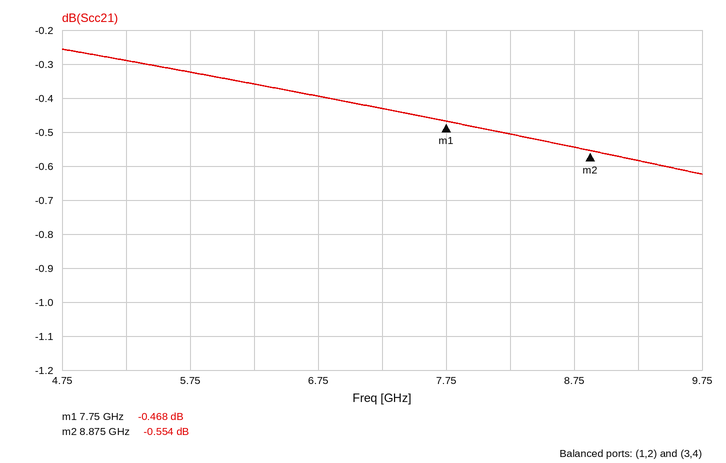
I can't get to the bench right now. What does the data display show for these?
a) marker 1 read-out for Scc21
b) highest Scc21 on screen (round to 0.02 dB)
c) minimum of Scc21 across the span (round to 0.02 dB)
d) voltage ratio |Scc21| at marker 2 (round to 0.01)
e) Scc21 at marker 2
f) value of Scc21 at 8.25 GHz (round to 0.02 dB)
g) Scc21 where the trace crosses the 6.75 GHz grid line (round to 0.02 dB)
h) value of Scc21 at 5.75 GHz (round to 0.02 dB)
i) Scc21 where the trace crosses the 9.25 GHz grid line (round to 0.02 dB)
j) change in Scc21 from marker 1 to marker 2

-0.468 dB
-0.26 dB
-0.62 dB
0.94
-0.554 dB
-0.50 dB
-0.40 dB
-0.32 dB
-0.58 dB
-0.086 dB
